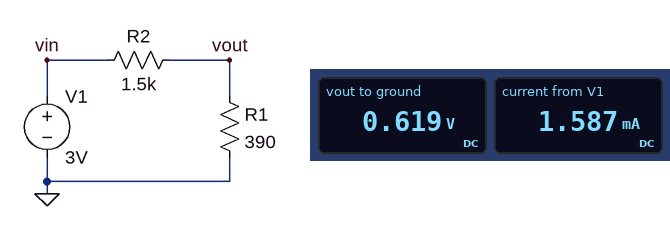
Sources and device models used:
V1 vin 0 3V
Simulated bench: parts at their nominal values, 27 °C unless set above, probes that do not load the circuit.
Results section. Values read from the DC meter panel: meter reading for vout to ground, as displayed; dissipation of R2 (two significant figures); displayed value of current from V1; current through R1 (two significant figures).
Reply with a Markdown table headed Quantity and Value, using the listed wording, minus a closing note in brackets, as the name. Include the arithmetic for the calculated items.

| Quantity | Value |
|---|---|
| meter reading for vout to ground, as displayed | 0.619 V |
| dissipation of R2 | (3 V - 619 mV)^2 / 1.5 kΩ = 3.8 mW |
| displayed value of current from V1 | 1.587 mA |
| current through R1 | (619 mV) / 390 Ω = 1.6 mA |
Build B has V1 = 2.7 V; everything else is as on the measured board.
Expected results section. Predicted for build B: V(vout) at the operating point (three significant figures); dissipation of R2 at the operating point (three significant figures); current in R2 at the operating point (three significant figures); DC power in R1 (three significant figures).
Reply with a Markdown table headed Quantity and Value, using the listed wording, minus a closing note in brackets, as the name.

| Quantity | Value |
|---|---|
| V(vout) at the operating point | 557 mV |
| dissipation of R2 at the operating point | 3.06 mW |
| current in R2 at the operating point | 1.43 mA |
| DC power in R1 | 796 µW |
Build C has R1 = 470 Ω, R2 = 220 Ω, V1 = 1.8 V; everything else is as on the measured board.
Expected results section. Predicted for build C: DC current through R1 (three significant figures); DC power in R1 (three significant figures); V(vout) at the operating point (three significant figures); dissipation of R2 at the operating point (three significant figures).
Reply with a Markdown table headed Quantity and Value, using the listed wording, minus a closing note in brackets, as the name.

| Quantity | Value |
|---|---|
| DC current through R1 | 2.61 mA |
| DC power in R1 | 3.20 mW |
| V(vout) at the operating point | 1.23 V |
| dissipation of R2 at the operating point | 1.50 mW |
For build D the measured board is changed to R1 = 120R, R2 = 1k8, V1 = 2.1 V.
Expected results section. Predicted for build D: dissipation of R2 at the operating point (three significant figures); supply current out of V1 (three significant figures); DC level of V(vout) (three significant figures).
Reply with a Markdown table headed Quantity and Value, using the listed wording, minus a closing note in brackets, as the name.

| Quantity | Value |
|---|---|
| dissipation of R2 at the operating point | 2.15 mW |
| supply current out of V1 | 1.09 mA |
| DC level of V(vout) | 131 mV |
